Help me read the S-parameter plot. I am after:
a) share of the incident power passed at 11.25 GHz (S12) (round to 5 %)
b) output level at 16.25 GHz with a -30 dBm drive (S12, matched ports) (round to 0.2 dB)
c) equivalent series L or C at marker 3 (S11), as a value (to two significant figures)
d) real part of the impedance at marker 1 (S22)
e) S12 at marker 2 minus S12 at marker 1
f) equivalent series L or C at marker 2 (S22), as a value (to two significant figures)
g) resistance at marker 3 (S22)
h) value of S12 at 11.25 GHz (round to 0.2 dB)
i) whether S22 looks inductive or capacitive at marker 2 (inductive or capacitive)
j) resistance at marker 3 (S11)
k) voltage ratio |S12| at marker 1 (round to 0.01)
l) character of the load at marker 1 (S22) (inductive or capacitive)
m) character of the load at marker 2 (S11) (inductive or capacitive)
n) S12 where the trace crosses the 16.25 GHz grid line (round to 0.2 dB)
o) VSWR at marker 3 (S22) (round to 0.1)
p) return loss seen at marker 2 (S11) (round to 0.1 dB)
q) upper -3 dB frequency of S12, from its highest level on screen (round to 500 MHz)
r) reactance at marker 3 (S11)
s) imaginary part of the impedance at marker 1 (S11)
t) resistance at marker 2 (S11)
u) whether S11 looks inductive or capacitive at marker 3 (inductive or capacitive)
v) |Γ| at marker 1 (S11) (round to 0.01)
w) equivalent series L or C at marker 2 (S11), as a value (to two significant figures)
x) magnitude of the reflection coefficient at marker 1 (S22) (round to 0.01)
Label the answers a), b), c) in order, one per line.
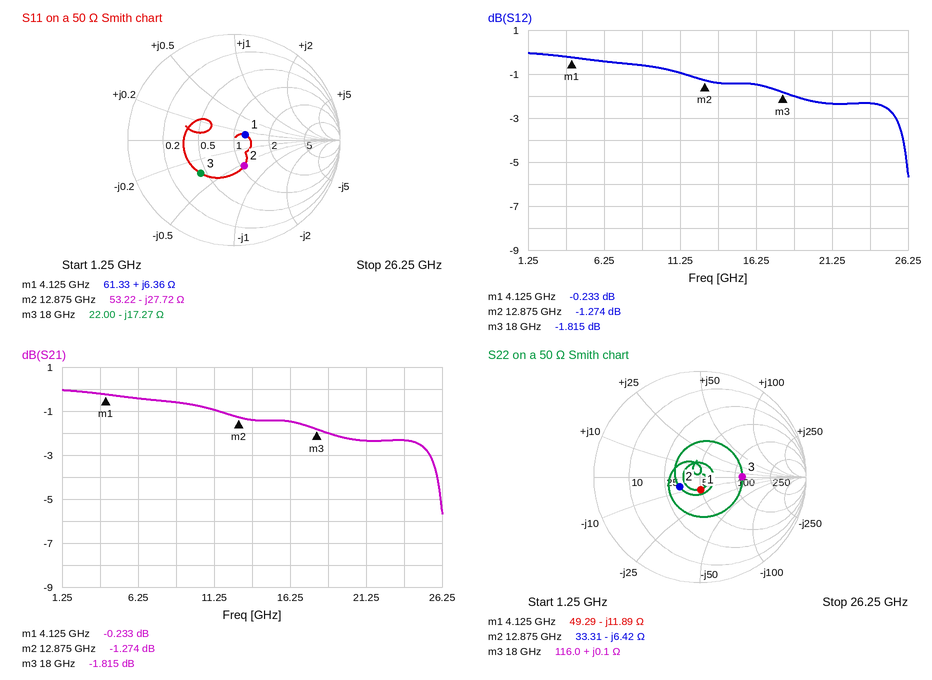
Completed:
a) 80 %
b) -31.4 dBm
c) 510 fF
d) 49.29 Ω
e) -1.041 dB
f) 1.9 pF
g) 116.0 Ω
h) -1.0 dB
i) capacitive
j) 22.00 Ω
k) 0.97
l) capacitive
m) capacitive
n) -1.4 dB
o) 2.3
p) 11.7 dB
q) 25.5 GHz
r) -17.27 Ω
s) +6.36 Ω
t) 53.22 Ω
u) capacitive
v) 0.12
w) 450 fF
x) 0.12
